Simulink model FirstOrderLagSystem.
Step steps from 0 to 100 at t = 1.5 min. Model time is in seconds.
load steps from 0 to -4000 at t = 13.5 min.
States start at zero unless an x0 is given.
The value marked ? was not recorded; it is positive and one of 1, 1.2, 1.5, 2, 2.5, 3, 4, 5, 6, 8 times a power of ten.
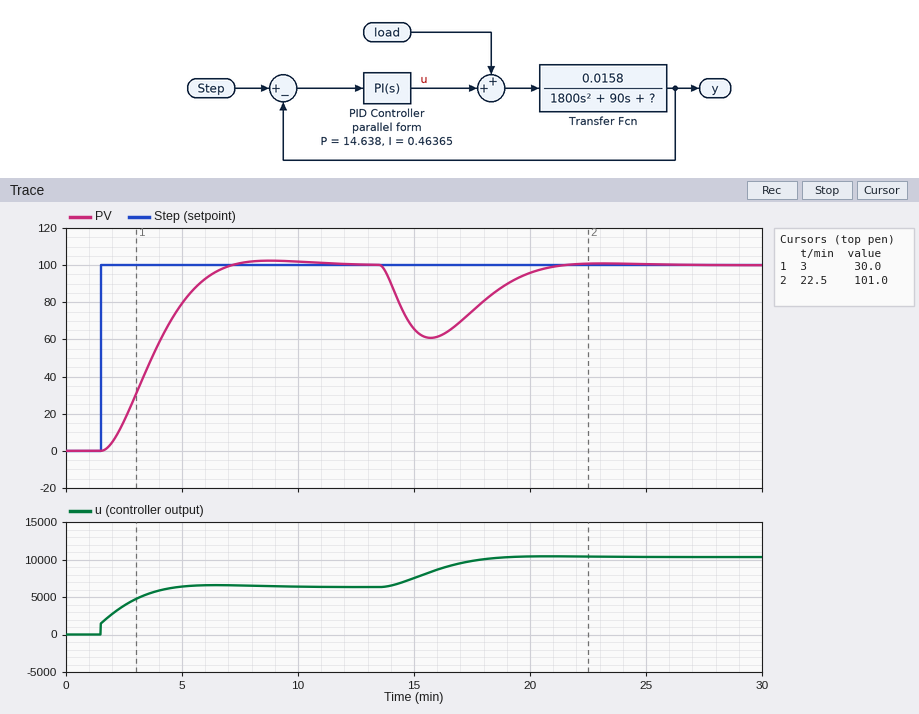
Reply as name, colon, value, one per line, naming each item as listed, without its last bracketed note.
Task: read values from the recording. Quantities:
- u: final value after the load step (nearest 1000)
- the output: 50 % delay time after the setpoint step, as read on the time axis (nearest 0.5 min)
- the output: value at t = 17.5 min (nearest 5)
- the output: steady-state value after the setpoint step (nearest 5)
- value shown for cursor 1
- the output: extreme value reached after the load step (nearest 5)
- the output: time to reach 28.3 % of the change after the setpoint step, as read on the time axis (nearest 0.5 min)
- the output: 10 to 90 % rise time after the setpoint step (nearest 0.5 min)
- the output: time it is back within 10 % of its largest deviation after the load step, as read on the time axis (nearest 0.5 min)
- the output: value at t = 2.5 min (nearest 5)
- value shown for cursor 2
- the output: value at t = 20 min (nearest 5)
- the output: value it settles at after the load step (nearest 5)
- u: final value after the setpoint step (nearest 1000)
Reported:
u: final value after the load step: 10000
the output: 50 % delay time after the setpoint step, as read on the time axis: 3.5 min
the output: value at t = 17.5 min: 75
the output: steady-state value after the setpoint step: 100
value shown for cursor 1: 30.0
the output: extreme value reached after the load step: 60
the output: time to reach 28.3 % of the change after the setpoint step, as read on the time axis: 3.0 min
the output: 10 to 90 % rise time after the setpoint step: 3.5 min
the output: time it is back within 10 % of its largest deviation after the load step, as read on the time axis: 20.0 min
the output: value at t = 2.5 min: 15
value shown for cursor 2: 101.0
the output: value at t = 20 min: 95
the output: value it settles at after the load step: 100
u: final value after the setpoint step: 6000
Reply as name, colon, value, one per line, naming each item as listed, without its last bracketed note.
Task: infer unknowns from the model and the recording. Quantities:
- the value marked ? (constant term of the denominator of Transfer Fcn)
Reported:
the value marked ?: 1
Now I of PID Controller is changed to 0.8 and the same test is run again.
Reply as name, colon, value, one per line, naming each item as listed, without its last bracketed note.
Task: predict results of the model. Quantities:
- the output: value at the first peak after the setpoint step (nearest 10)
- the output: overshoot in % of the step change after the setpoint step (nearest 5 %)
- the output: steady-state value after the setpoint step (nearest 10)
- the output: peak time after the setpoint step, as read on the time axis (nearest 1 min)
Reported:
the output: value at the first peak after the setpoint step: 120
the output: overshoot in % of the step change after the setpoint step: 15 %
the output: steady-state value after the setpoint step: 100
the output: peak time after the setpoint step, as read on the time axis: 6 min
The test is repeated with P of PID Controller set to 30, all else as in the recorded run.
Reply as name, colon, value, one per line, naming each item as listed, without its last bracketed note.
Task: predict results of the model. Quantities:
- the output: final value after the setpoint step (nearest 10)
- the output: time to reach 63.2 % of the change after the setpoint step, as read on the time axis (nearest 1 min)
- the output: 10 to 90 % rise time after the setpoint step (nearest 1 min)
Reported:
the output: final value after the setpoint step: 100
the output: time to reach 63.2 % of the change after the setpoint step, as read on the time axis: 4 min
the output: 10 to 90 % rise time after the setpoint step: 4 min
